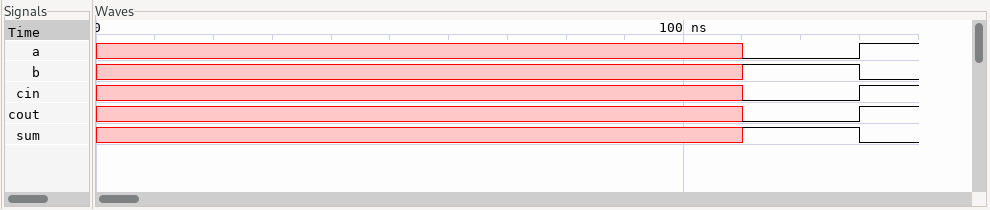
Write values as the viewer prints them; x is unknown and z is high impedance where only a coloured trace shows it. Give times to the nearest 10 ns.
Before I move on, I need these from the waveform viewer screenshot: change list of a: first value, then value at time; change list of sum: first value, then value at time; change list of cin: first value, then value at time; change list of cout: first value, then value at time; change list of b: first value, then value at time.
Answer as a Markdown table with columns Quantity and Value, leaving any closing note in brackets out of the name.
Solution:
| Quantity | Value |
|---|---|
| change list of a: first value, then value at time | x, 0 at 110 ns, 1 at 130 ns |
| change list of sum: first value, then value at time | x, 1 at 110 ns, 0 at 130 ns |
| change list of cin: first value, then value at time | x, 0 at 110 ns, 1 at 130 ns |
| change list of cout: first value, then value at time | x, 0 at 110 ns, 1 at 130 ns |
| change list of b: first value, then value at time | x, 1 at 110 ns, 0 at 130 ns |
